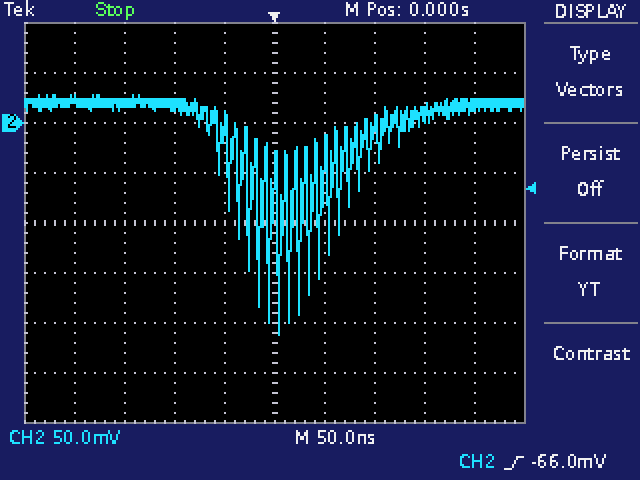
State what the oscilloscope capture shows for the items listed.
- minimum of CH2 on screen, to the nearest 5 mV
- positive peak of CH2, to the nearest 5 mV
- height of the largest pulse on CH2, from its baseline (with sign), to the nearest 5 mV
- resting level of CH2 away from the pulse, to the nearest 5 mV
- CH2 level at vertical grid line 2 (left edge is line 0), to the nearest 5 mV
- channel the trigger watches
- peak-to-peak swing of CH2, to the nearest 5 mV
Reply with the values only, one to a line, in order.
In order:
-210 mV
30 mV
-230 mV
20 mV
20 mV
CH2
240 mV
